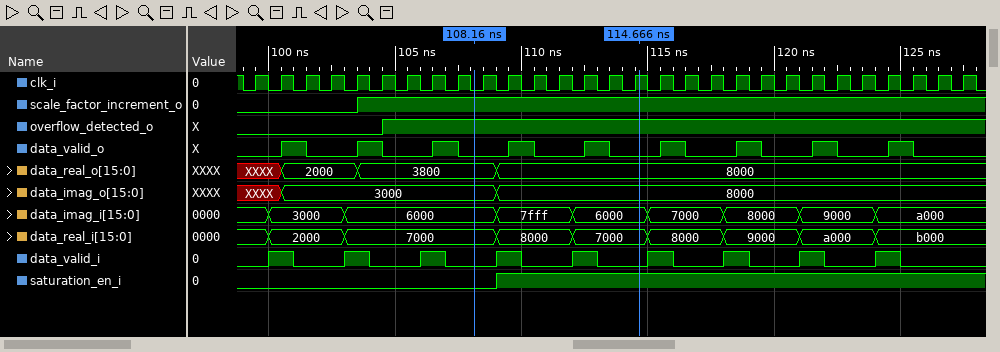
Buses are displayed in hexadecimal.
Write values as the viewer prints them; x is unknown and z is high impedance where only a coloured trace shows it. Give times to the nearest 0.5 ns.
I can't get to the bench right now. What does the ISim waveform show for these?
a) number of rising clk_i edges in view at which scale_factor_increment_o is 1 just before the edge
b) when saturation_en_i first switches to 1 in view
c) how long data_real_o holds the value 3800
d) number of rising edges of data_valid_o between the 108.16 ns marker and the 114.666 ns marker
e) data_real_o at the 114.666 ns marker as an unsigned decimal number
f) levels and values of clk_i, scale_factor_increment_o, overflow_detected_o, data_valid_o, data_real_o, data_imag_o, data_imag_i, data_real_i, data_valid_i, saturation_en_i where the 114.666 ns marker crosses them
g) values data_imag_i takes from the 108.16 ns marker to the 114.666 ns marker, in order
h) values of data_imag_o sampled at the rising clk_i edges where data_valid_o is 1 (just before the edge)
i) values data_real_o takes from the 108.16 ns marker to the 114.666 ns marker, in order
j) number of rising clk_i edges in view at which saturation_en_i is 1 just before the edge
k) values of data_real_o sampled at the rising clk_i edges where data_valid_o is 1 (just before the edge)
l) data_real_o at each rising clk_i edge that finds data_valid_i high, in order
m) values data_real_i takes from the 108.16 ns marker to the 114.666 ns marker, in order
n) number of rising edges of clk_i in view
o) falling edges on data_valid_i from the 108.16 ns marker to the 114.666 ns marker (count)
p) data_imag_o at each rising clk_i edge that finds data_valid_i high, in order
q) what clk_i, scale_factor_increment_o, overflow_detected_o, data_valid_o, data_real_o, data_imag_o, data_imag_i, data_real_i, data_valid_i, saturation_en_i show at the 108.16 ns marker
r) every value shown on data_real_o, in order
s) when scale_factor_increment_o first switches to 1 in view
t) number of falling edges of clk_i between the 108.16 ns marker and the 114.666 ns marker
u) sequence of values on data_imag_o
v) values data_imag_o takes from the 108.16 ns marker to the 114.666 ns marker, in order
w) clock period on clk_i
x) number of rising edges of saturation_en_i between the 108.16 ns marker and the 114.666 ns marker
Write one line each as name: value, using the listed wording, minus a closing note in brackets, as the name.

number of rising clk_i edges in view at which scale_factor_increment_o is 1 just before the edge: 24
when saturation_en_i first switches to 1 in view: 109 ns
how long data_real_o holds the value 3800: 5.5 ns
number of rising edges of data_valid_o between the 108.16 ns marker and the 114.666 ns marker: 2
data_real_o at the 114.666 ns marker as an unsigned decimal number: 32768
levels and values of clk_i, scale_factor_increment_o, overflow_detected_o, data_valid_o, data_real_o, data_imag_o, data_imag_i, data_real_i, data_valid_i, saturation_en_i where the 114.666 ns marker crosses them: clk_i=1, scale_factor_increment_o=1, overflow_detected_o=1, data_valid_o=0, data_real_o=8000, data_imag_o=8000, data_imag_i=6000, data_real_i=7000, data_valid_i=0, saturation_en_i=1
values data_imag_i takes from the 108.16 ns marker to the 114.666 ns marker, in order: 6000, 7fff, 6000
values of data_imag_o sampled at the rising clk_i edges where data_valid_o is 1: 3000, 3000, 3000, 8000, 8000, 8000, 8000, 8000, 8000
values data_real_o takes from the 108.16 ns marker to the 114.666 ns marker, in order: 3800, 8000
number of rising clk_i edges in view at which saturation_en_i is 1 just before the edge: 19
values of data_real_o sampled at the rising clk_i edges where data_valid_o is 1: 2000, 3800, 3800, 8000, 8000, 8000, 8000, 8000, 8000
data_real_o at each rising clk_i edge that finds data_valid_i high, in order: XXXX, 2000, 3800, 8000, 8000, 8000, 8000, 8000, 8000
values data_real_i takes from the 108.16 ns marker to the 114.666 ns marker, in order: 7000, 8000, 7000
number of rising edges of clk_i in view: 29
falling edges on data_valid_i from the 108.16 ns marker to the 114.666 ns marker: 2
data_imag_o at each rising clk_i edge that finds data_valid_i high, in order: XXXX, 3000, 3000, 8000, 8000, 8000, 8000, 8000, 8000
what clk_i, scale_factor_increment_o, overflow_detected_o, data_valid_o, data_real_o, data_imag_o, data_imag_i, data_real_i, data_valid_i, saturation_en_i show at the 108.16 ns marker: clk_i=0, scale_factor_increment_o=1, overflow_detected_o=1, data_valid_o=0, data_real_o=3800, data_imag_o=3000, data_imag_i=6000, data_real_i=7000, data_valid_i=0, saturation_en_i=0
every value shown on data_real_o, in order: XXXX, 2000, 3800, 8000
when scale_factor_increment_o first switches to 1 in view: 103.5 ns
number of falling edges of clk_i between the 108.16 ns marker and the 114.666 ns marker: 6
sequence of values on data_imag_o: XXXX, 3000, 8000
values data_imag_o takes from the 108.16 ns marker to the 114.666 ns marker, in order: 3000, 8000
clock period on clk_i: 1 ns
number of rising edges of saturation_en_i between the 108.16 ns marker and the 114.666 ns marker: 1
